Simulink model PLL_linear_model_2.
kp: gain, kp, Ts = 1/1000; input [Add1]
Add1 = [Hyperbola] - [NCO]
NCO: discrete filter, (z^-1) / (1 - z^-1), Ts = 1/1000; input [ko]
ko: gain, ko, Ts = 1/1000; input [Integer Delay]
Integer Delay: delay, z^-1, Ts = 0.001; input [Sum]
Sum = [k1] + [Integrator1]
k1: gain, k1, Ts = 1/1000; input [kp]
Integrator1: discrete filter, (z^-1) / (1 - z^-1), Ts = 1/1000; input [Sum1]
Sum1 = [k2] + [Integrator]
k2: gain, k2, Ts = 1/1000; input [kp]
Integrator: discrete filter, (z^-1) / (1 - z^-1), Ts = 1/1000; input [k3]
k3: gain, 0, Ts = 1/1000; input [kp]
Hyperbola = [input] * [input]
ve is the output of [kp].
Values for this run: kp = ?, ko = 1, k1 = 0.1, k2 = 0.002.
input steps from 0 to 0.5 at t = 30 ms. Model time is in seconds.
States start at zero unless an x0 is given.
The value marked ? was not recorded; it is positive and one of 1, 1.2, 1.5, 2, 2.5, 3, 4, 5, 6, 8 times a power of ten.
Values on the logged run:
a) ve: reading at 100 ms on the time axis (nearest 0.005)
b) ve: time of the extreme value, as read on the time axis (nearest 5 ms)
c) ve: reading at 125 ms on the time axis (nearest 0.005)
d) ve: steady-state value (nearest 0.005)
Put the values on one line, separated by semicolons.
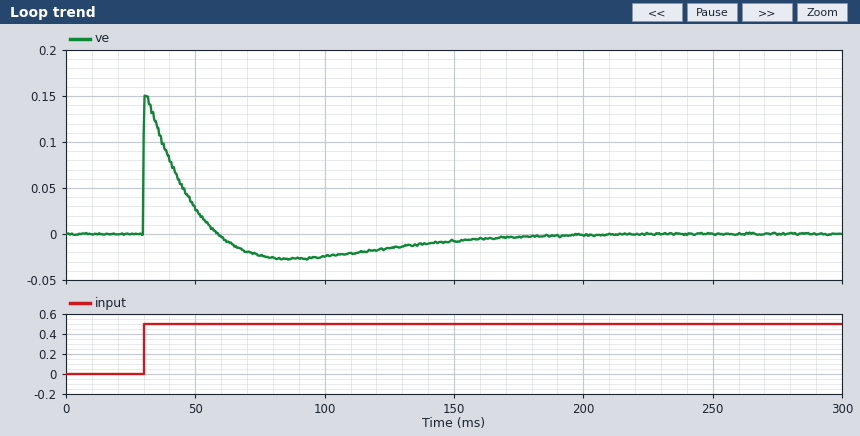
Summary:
-0.025; 30 ms; -0.015; 0.000
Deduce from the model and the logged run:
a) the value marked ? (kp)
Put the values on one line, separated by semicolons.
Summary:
0.6
